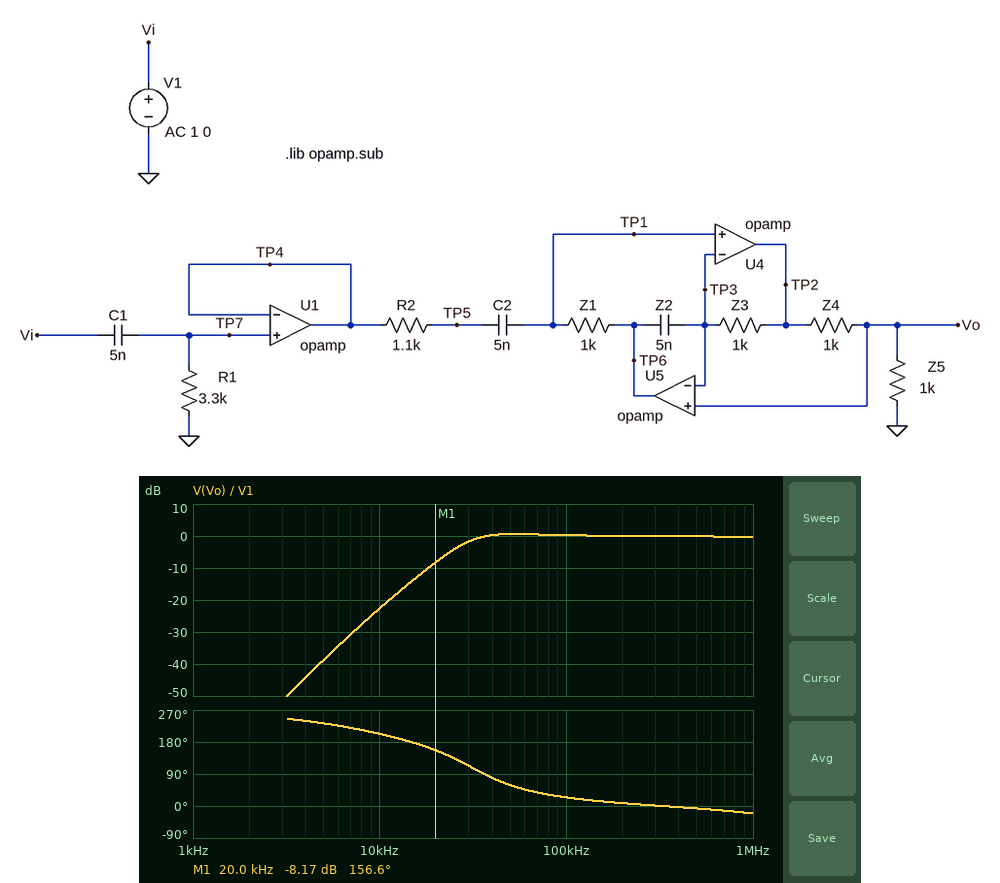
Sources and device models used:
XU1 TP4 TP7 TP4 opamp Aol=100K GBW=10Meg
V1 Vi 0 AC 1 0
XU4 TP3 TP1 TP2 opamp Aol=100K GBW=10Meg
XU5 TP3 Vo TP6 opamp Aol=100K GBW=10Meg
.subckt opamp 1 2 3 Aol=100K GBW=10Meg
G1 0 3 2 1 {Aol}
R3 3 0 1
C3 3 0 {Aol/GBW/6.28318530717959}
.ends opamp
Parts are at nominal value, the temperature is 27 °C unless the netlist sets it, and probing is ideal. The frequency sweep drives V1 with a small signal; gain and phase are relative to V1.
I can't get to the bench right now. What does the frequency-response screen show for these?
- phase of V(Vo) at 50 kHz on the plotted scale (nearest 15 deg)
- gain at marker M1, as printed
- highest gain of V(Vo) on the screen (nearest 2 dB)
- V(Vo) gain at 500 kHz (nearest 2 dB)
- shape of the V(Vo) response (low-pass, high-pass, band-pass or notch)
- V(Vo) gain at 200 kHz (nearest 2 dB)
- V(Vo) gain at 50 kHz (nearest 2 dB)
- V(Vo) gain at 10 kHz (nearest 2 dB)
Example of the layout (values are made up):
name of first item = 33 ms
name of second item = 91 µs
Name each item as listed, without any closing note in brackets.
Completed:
phase of V(Vo) at 50 kHz on the plotted scale = 60 deg
gain at marker M1, as printed = -8.17 dB
highest gain of V(Vo) on the screen = 0 dB
V(Vo) gain at 500 kHz = 0 dB
shape of the V(Vo) response = high-pass
V(Vo) gain at 200 kHz = 0 dB
V(Vo) gain at 50 kHz = 0 dB
V(Vo) gain at 10 kHz = -22 dB
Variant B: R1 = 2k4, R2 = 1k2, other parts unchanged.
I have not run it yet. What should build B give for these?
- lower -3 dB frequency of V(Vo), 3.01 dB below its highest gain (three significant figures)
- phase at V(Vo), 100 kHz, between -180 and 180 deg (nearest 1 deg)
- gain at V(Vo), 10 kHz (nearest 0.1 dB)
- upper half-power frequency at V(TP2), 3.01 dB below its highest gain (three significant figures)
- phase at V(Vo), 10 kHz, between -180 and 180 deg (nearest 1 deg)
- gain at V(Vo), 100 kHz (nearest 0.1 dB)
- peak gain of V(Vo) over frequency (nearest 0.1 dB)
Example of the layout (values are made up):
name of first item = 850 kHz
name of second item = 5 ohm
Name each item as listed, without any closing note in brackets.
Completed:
lower -3 dB frequency of V(Vo), 3.01 dB below its highest gain = 30.0 kHz
phase at V(Vo), 100 kHz, between -180 and 180 deg = 28 deg
gain at V(Vo), 10 kHz = -24.3 dB
upper half-power frequency at V(TP2), 3.01 dB below its highest gain = 2.76 MHz
phase at V(Vo), 10 kHz, between -180 and 180 deg = -150 deg
gain at V(Vo), 100 kHz = 0.1 dB
peak gain of V(Vo) over frequency = 0.2 dB
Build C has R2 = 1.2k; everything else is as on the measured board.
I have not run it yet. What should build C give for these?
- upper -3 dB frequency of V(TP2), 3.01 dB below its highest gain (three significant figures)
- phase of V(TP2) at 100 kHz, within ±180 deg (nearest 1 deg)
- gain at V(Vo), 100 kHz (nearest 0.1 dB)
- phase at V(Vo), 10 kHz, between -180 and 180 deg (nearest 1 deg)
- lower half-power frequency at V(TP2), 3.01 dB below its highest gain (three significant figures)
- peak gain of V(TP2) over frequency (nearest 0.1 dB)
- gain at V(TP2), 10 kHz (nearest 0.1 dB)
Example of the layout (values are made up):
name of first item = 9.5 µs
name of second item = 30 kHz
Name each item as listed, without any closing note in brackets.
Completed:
upper -3 dB frequency of V(TP2), 3.01 dB below its highest gain = 2.71 MHz
phase of V(TP2) at 100 kHz, within ±180 deg = 26 deg
gain at V(Vo), 100 kHz = 0.2 dB
phase at V(Vo), 10 kHz, between -180 and 180 deg = -159 deg
lower half-power frequency at V(TP2), 3.01 dB below its highest gain = 29.3 kHz
peak gain of V(TP2) over frequency = 6.3 dB
gain at V(TP2), 10 kHz = -16.7 dB
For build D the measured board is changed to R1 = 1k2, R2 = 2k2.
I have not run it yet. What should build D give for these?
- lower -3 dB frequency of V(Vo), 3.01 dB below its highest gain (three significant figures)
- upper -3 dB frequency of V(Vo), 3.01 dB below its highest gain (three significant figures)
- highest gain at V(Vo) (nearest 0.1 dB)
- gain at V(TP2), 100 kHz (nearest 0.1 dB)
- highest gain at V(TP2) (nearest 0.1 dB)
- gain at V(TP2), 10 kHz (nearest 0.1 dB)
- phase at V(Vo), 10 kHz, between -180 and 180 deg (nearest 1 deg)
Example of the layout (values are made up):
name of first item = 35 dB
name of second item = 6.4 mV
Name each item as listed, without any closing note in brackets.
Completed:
lower -3 dB frequency of V(Vo), 3.01 dB below its highest gain = 63.1 kHz
upper -3 dB frequency of V(Vo), 3.01 dB below its highest gain = 1.92 MHz
highest gain at V(Vo) = -0.1 dB
gain at V(TP2), 100 kHz = 4.7 dB
highest gain at V(TP2) = 5.9 dB
gain at V(TP2), 10 kHz = -24.2 dB
phase at V(Vo), 10 kHz, between -180 and 180 deg = -148 deg
